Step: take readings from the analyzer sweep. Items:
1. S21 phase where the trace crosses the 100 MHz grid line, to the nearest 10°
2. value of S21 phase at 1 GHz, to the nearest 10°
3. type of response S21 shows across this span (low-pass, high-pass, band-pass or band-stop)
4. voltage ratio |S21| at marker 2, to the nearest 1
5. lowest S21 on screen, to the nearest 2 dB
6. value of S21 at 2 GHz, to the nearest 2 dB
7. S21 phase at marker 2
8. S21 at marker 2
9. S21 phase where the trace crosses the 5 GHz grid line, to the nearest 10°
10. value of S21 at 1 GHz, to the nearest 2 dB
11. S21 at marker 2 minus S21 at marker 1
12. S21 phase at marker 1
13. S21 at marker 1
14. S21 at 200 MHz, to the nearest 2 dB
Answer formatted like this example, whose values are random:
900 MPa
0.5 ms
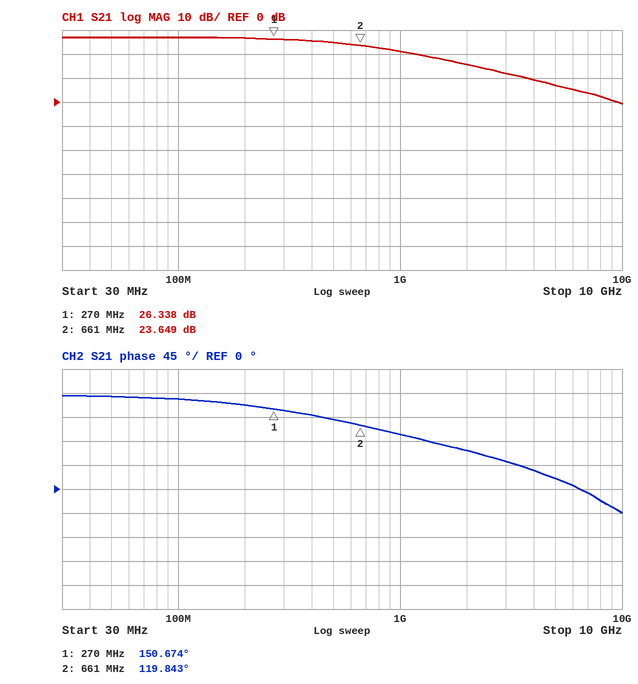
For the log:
170°
100°
low-pass
15
0 dB
16 dB
119.843°
23.649 dB
20°
22 dB
-2.689 dB
150.674°
26.338 dB
26 dB
